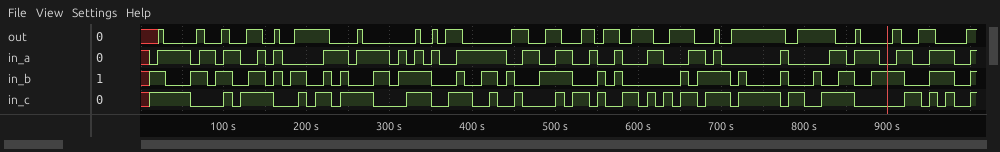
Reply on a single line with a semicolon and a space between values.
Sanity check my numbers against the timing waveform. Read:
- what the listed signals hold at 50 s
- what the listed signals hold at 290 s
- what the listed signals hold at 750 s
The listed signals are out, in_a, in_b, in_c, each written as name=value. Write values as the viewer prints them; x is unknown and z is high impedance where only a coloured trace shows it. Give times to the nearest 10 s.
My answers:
out=0, in_a=1, in_b=0, in_c=1; out=0, in_a=1, in_b=1, in_c=0; out=1, in_a=0, in_b=0, in_c=1
